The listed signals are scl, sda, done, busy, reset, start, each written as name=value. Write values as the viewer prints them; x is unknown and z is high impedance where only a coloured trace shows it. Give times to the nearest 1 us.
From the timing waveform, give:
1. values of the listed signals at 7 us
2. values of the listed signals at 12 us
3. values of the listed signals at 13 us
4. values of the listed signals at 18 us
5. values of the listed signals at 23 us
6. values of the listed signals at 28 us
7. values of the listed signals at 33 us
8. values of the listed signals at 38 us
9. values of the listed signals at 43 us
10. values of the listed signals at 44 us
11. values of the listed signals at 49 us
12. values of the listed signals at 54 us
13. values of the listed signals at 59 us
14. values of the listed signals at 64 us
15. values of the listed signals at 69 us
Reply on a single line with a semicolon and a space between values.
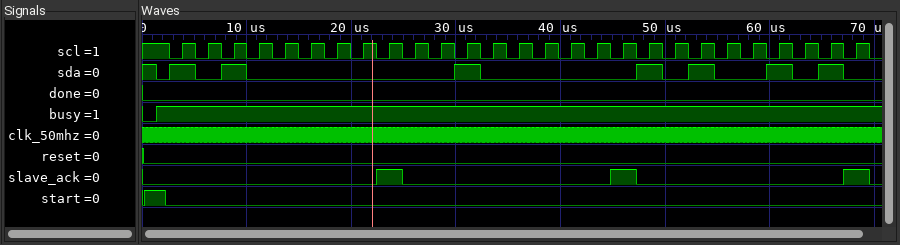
scl=1, sda=0, done=0, busy=1, reset=0, start=0; scl=1, sda=0, done=0, busy=1, reset=0, start=0; scl=0, sda=0, done=0, busy=1, reset=0, start=0; scl=0, sda=0, done=0, busy=1, reset=0, start=0; scl=0, sda=0, done=0, busy=1, reset=0, start=0; scl=0, sda=0, done=0, busy=1, reset=0, start=0; scl=0, sda=0, done=0, busy=1, reset=0, start=0; scl=0, sda=0, done=0, busy=1, reset=0, start=0; scl=0, sda=0, done=0, busy=1, reset=0, start=0; scl=1, sda=0, done=0, busy=1, reset=0, start=0; scl=1, sda=1, done=0, busy=1, reset=0, start=0; scl=1, sda=1, done=0, busy=1, reset=0, start=0; scl=1, sda=0, done=0, busy=1, reset=0, start=0; scl=1, sda=0, done=0, busy=1, reset=0, start=0; scl=1, sda=0, done=0, busy=1, reset=0, start=0
